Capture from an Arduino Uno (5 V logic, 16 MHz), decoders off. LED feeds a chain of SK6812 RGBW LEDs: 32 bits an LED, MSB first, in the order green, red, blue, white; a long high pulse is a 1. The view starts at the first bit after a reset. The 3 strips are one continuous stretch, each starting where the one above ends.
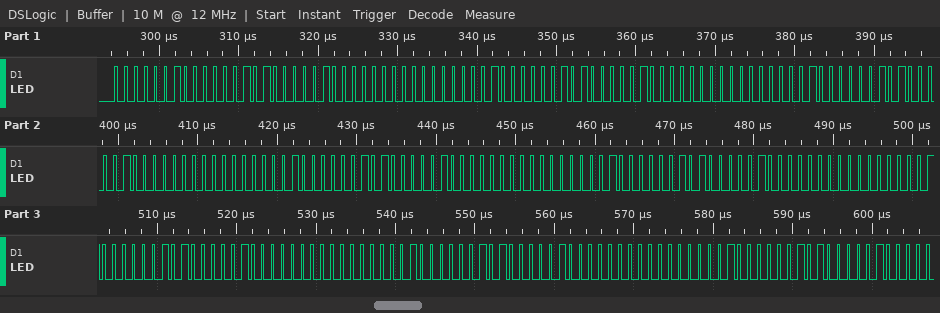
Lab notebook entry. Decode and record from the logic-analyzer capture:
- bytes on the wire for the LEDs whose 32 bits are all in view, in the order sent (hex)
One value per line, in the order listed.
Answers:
02 05 04 00 02 05 04 00 02 05 04 00 02 05 04 00 02 05 04 00 02 05 04 00 02 05 04 00
